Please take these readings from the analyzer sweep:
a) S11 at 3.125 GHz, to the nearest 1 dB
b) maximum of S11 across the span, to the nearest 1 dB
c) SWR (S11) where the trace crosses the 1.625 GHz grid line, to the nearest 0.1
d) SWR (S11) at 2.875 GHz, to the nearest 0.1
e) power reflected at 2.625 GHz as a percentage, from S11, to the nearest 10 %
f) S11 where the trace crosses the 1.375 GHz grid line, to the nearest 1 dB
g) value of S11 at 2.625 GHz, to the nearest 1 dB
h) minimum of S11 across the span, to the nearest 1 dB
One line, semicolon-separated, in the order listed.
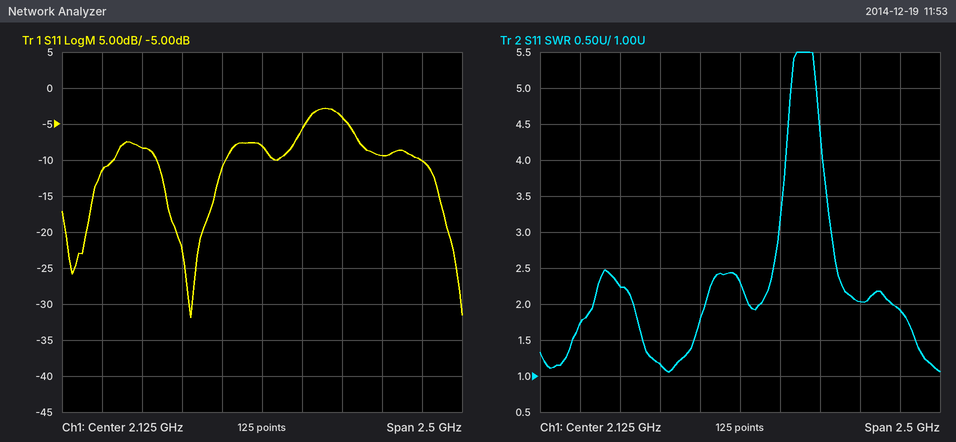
-10 dB; -3 dB; 1.2; 2.0; 40 %; -8 dB; -4 dB; -32 dB
